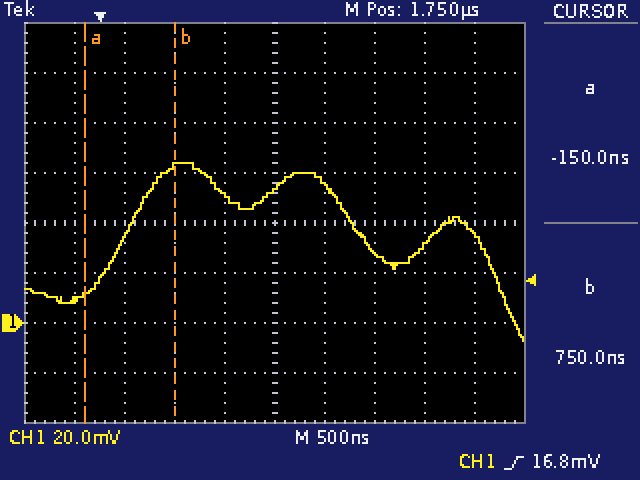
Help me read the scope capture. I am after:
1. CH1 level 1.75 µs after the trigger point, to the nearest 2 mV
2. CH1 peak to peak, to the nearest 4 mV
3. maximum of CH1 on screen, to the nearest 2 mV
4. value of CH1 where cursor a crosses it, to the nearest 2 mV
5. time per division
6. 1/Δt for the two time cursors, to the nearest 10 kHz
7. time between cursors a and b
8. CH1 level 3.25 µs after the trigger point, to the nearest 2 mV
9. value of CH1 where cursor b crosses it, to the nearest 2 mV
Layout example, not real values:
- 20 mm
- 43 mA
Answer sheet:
- 54 mV
- 72 mV
- 64 mV
- 12 mV
- 500 ns
- 1.11 MHz
- 900 ns
- 32 mV
- 62 mV
